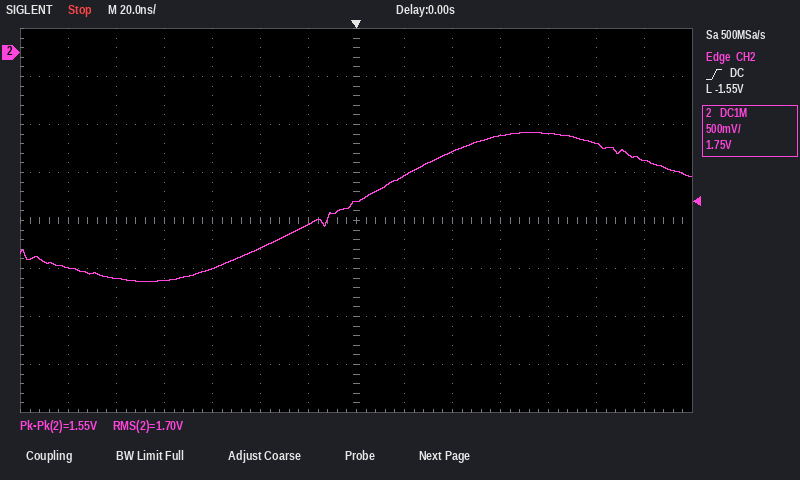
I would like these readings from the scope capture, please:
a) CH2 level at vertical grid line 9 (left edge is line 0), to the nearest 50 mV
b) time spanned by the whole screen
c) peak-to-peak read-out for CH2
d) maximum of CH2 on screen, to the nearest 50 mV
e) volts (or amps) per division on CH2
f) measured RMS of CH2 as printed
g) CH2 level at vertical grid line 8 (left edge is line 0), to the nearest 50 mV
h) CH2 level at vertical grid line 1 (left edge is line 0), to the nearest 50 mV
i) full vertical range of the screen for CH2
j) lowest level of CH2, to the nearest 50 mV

-1.05 V
280 ns
1.55 V
-850 mV
500 mV
1.70 V
-1.30 V
-2.25 V
4 V
-2.40 V
